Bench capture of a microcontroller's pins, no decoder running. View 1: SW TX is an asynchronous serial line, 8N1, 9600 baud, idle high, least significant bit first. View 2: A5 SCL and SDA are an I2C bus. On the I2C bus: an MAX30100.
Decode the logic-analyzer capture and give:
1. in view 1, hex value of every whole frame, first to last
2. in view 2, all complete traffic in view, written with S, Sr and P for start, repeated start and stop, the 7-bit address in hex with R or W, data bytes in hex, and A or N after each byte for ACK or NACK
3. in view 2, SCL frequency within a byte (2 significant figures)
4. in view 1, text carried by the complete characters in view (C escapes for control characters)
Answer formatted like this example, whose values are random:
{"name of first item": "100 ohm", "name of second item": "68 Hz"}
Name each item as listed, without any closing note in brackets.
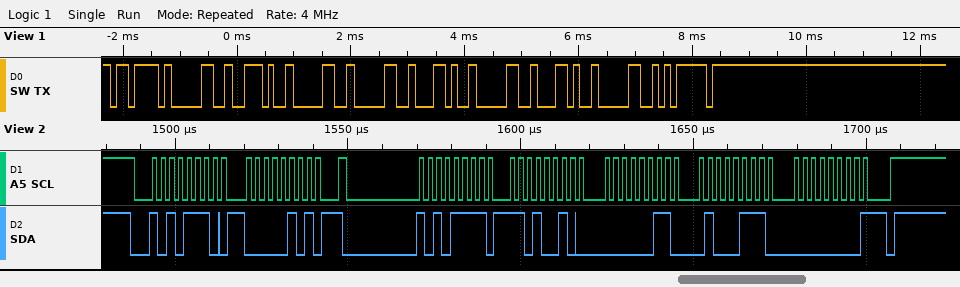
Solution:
{"in view 1, hex value of every whole frame, first to last": "7B 30 2E 30 30 2C 30 2C 30 7D", "in view 2, all complete traffic in view, written with S, Sr and P for start, repeated start and stop, the 7-bit address in hex with R or W, data bytes in hex, and A or N after each byte for ACK or NACK": "S 57W A 05 A Sr 57R A D2 A 03 A 47 A 00 N P", "in view 2, SCL frequency within a byte": "400 kHz", "in view 1, text carried by the complete characters in view": "\"{0.00,0,0}\""}
